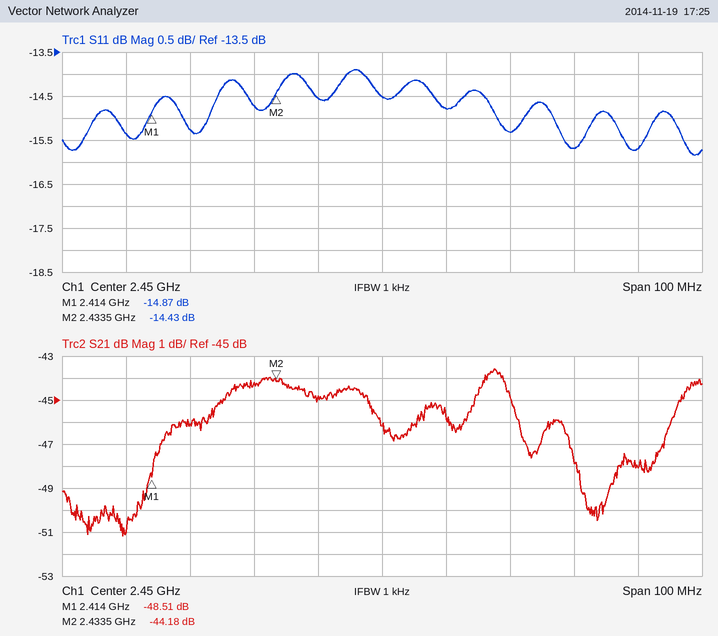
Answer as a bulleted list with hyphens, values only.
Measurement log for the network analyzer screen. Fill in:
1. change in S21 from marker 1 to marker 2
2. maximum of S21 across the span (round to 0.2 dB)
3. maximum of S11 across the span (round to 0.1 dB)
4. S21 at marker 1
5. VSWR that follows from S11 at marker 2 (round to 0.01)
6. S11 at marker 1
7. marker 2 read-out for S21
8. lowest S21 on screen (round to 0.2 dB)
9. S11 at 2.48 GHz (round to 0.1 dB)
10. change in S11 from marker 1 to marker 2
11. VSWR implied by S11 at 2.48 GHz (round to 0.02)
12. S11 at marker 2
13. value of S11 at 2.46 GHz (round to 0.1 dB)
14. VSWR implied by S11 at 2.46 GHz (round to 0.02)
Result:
- 4.33 dB
- -43.6 dB
- -13.9 dB
- -48.51 dB
- 1.47
- -14.87 dB
- -44.18 dB
- -51.2 dB
- -15.7 dB
- 0.44 dB
- 1.40
- -14.43 dB
- -14.8 dB
- 1.44
